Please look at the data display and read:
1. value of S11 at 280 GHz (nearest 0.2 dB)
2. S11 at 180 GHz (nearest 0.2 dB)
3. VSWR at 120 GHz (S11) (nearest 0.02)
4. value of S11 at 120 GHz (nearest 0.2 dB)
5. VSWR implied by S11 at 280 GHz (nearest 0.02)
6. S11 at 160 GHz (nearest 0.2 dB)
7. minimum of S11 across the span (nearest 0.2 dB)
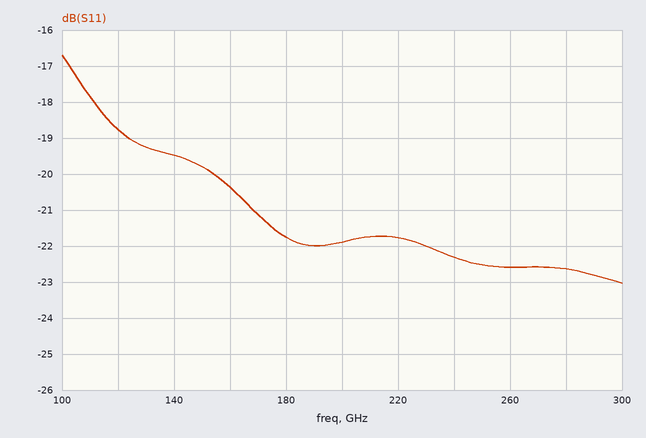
-22.6 dB
-21.8 dB
1.26
-18.8 dB
1.16
-20.4 dB
-23.0 dB
